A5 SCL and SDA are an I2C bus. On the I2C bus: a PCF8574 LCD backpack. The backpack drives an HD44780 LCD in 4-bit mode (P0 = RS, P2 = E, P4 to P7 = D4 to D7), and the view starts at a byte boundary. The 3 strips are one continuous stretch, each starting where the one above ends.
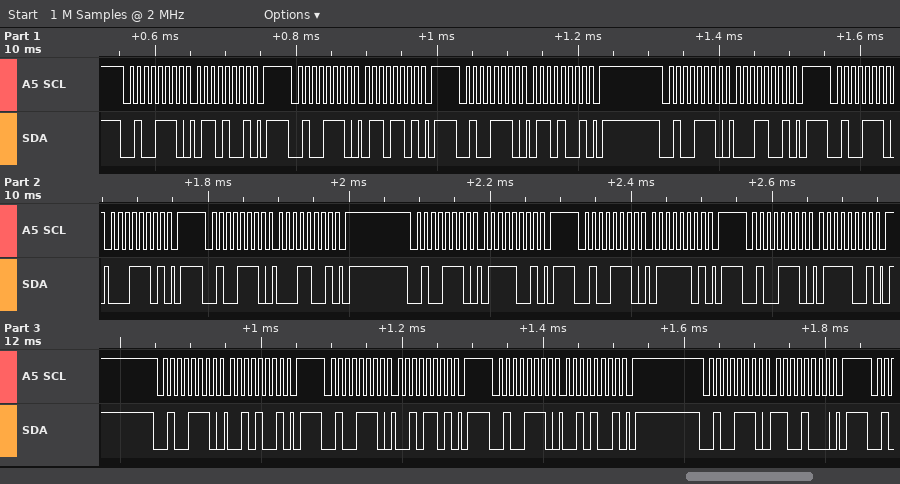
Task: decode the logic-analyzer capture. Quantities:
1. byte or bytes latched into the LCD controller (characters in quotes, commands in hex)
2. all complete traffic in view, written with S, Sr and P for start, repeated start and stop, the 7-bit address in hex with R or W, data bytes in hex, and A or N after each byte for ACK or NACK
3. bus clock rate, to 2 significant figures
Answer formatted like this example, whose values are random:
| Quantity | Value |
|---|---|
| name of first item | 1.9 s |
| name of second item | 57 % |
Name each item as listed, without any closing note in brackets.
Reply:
| Quantity | Value |
|---|---|
| byte or bytes latched into the LCD controller | 'a' 'r' |
| all complete traffic in view, written with S, Sr and P for start, repeated start and stop, the 7-bit address in hex with R or W, data bytes in hex, and A or N after each byte for ACK or NACK | S 27W A 69 A P S 27W A 6D A P S 27W A 69 A P S 27W A 19 A P S 27W A 1D A P S 27W A 19 A P S 27W A 79 A P S 27W A 7D A P S 27W A 79 A P S 27W A 29 A P S 27W A 2D A P S 27W A 29 A P S 27W A C8 A P |
| bus clock rate, to 2 significant figures | 100 kHz |
